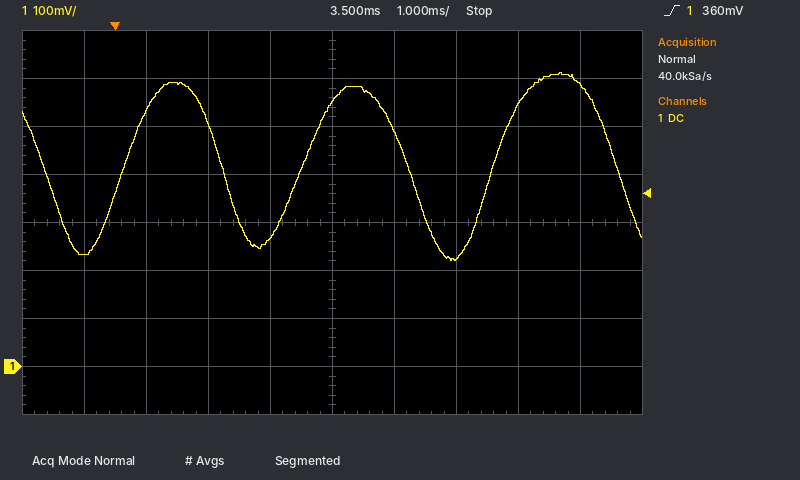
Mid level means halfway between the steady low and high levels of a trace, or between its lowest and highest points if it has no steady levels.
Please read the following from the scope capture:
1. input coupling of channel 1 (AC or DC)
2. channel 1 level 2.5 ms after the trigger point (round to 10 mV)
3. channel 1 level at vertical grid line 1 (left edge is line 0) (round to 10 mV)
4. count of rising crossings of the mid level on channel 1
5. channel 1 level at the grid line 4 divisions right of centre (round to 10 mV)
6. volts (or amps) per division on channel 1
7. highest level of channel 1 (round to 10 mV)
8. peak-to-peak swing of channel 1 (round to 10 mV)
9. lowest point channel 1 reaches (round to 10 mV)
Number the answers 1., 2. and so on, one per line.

1. DC
2. 270 mV
3. 230 mV
4. 3
5. 590 mV
6. 100 mV
7. 610 mV
8. 390 mV
9. 220 mV
